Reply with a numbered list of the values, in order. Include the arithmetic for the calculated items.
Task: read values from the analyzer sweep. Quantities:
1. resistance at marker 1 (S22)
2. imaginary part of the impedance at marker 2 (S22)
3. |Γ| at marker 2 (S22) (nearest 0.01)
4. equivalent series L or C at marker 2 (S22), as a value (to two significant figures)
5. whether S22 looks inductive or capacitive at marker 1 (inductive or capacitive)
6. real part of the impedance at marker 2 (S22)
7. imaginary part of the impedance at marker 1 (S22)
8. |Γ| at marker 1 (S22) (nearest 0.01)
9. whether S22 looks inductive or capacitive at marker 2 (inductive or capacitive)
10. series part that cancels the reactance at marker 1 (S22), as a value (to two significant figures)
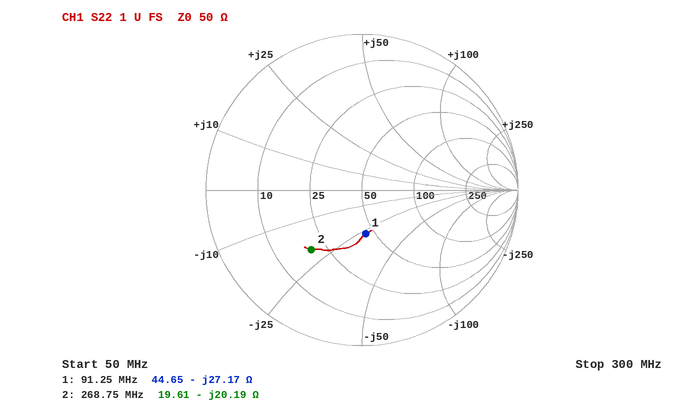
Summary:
1. 44.65 Ω
2. -20.19 Ω
3. 0.50
4. C = 1/(2π × 268.75 MHz × 20.19 Ω) ≈ 29 pF
5. capacitive
6. 19.61 Ω
7. -27.17 Ω
8. 0.28
9. capacitive
10. L = 27.17 Ω/(2π × 91.25 MHz) ≈ 47 nH
